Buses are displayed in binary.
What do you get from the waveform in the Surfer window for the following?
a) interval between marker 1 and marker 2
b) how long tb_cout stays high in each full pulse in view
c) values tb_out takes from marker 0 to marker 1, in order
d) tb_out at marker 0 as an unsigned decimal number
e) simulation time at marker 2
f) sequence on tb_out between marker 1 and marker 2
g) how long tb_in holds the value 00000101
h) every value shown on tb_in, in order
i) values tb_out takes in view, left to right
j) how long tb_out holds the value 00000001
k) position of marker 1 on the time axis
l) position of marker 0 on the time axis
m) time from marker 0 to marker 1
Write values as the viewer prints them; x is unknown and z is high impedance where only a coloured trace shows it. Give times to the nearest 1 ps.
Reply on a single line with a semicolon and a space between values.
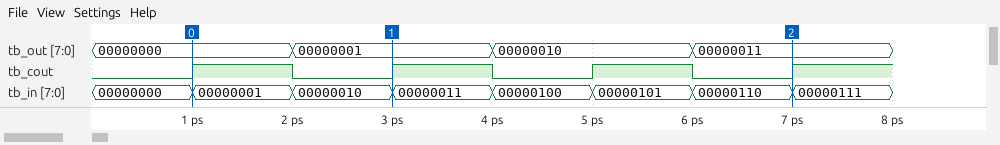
4 ps; 1 ps, 1 ps, 1 ps; 00000000, 00000001; 0; 7 ps; 00000001, 00000010, 00000011; 1 ps; 00000000, 00000001, 00000010, 00000011, 00000100, 00000101, 00000110, 00000111; 00000000, 00000001, 00000010, 00000011; 2 ps; 3 ps; 1 ps; 2 ps
